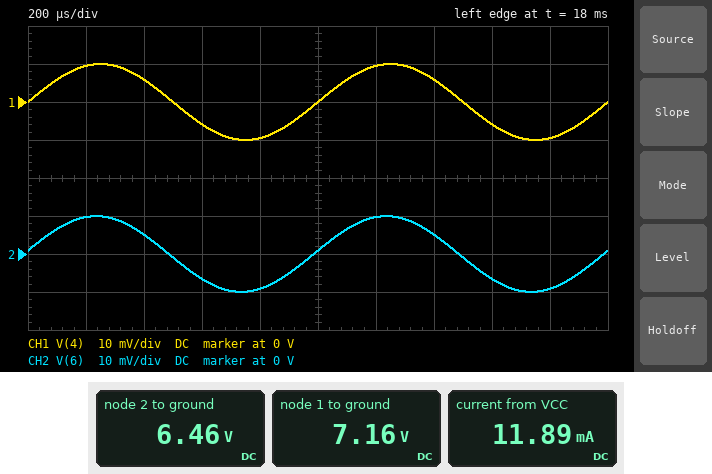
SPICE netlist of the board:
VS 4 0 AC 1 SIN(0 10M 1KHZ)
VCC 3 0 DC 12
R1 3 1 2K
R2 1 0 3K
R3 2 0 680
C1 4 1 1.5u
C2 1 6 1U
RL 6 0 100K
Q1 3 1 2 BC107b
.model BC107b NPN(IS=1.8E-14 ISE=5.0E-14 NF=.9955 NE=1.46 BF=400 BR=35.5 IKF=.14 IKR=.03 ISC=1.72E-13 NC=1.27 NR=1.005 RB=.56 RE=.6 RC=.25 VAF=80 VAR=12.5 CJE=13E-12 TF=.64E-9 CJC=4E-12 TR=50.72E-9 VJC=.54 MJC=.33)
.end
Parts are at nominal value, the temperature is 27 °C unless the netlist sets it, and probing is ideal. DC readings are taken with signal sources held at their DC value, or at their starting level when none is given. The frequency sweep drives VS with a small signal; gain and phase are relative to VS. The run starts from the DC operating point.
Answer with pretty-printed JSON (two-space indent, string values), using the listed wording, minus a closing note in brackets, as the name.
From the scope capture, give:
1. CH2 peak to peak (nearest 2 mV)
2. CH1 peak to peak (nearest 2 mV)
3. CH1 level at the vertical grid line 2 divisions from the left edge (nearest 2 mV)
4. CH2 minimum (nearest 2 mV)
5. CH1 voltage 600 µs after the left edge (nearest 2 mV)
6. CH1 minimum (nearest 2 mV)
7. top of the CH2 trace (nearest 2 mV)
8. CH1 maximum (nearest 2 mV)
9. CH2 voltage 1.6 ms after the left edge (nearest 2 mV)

{
  "CH2 peak to peak": "20 mV",
  "CH1 peak to peak": "20 mV",
  "CH1 level at the vertical grid line 2 divisions from the left edge": "6 mV",
  "CH2 minimum": "-10 mV",
  "CH1 voltage 600 µs after the left edge": "-6 mV",
  "CH1 minimum": "-10 mV",
  "top of the CH2 trace": "10 mV",
  "CH1 maximum": "10 mV",
  "CH2 voltage 1.6 ms after the left edge": "-6 mV"
}
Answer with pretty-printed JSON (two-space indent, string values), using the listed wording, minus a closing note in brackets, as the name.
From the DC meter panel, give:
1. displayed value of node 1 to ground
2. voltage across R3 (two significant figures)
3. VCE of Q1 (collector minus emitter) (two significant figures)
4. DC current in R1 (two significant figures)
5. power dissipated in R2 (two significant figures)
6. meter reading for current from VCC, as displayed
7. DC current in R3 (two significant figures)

{
  "displayed value of node 1 to ground": "7.16 V",
  "voltage across R3": "6.5 V",
  "VCE of Q1 (collector minus emitter)": "5.5 V",
  "DC current in R1": "2.4 mA",
  "power dissipated in R2": "17 mW",
  "meter reading for current from VCC, as displayed": "11.89 mA",
  "DC current in R3": "9.5 mA"
}
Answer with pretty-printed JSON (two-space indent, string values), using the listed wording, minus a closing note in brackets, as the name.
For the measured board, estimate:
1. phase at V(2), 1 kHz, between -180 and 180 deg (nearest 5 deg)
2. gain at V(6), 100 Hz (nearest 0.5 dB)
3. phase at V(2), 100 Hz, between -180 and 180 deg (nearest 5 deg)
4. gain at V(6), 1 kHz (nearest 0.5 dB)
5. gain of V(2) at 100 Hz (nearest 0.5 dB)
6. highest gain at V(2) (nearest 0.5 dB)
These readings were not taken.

{
  "phase at V(2), 1 kHz, between -180 and 180 deg": "5 deg",
  "gain at V(6), 100 Hz": "-2.5 dB",
  "phase at V(2), 100 Hz, between -180 and 180 deg": "40 deg",
  "gain at V(6), 1 kHz": "0 dB",
  "gain of V(2) at 100 Hz": "-2.5 dB",
  "highest gain at V(2)": "0 dB"
}
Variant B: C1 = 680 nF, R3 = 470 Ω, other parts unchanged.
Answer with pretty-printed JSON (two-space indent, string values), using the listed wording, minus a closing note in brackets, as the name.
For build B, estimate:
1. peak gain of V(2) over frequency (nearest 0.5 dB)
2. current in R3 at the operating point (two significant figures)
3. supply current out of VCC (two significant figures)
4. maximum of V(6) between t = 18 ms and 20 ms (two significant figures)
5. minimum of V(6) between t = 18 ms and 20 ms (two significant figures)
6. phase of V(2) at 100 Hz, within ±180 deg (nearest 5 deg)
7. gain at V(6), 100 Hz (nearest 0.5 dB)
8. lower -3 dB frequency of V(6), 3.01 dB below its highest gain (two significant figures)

{
  "peak gain of V(2) over frequency": "0 dB",
  "current in R3 at the operating point": "14 mA",
  "supply current out of VCC": "16 mA",
  "maximum of V(6) between t = 18 ms and 20 ms": "9.8 mV",
  "minimum of V(6) between t = 18 ms and 20 ms": "-9.8 mV",
  "phase of V(2) at 100 Hz, within ±180 deg": "65 deg",
  "gain at V(6), 100 Hz": "-7.0 dB",
  "lower -3 dB frequency of V(6), 3.01 dB below its highest gain": "200 Hz"
}
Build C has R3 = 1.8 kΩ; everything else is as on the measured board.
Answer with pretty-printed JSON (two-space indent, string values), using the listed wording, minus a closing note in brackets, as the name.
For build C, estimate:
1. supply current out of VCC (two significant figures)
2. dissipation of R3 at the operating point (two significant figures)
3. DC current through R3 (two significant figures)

{
  "supply current out of VCC": "6.0 mA",
  "dissipation of R3 at the operating point": "24 mW",
  "DC current through R3": "3.6 mA"
}
